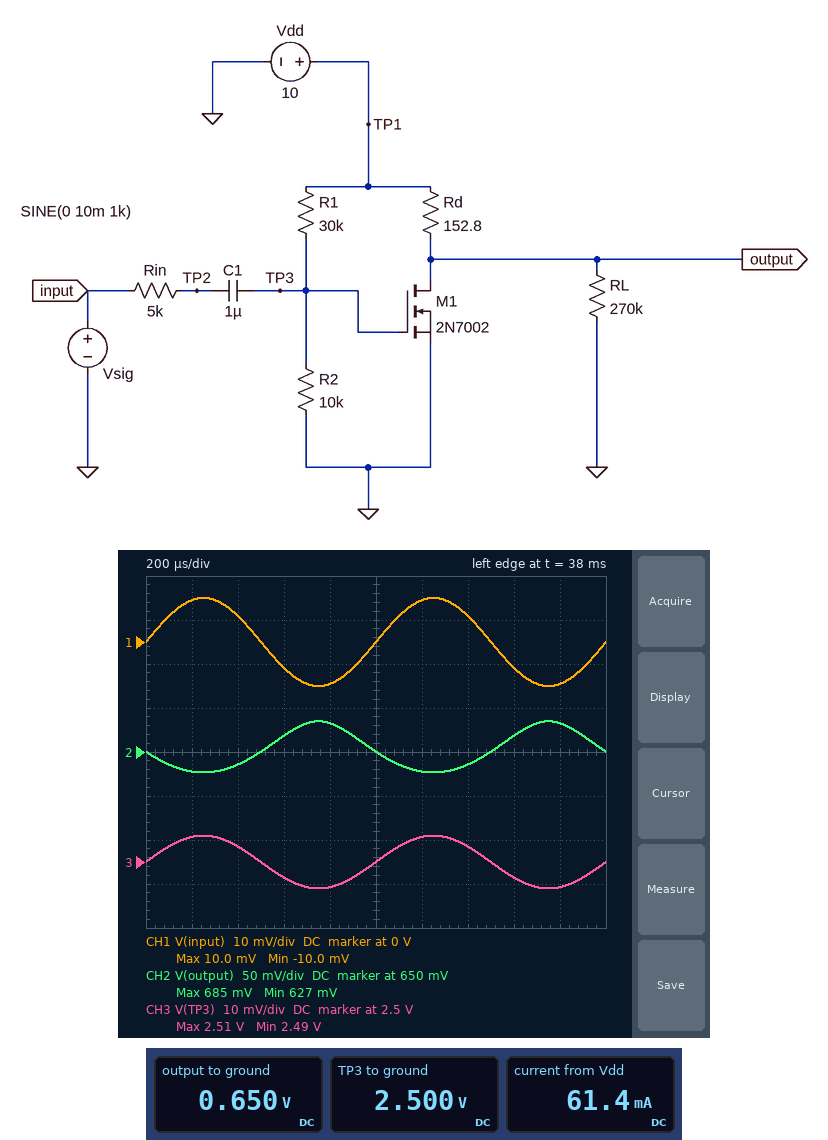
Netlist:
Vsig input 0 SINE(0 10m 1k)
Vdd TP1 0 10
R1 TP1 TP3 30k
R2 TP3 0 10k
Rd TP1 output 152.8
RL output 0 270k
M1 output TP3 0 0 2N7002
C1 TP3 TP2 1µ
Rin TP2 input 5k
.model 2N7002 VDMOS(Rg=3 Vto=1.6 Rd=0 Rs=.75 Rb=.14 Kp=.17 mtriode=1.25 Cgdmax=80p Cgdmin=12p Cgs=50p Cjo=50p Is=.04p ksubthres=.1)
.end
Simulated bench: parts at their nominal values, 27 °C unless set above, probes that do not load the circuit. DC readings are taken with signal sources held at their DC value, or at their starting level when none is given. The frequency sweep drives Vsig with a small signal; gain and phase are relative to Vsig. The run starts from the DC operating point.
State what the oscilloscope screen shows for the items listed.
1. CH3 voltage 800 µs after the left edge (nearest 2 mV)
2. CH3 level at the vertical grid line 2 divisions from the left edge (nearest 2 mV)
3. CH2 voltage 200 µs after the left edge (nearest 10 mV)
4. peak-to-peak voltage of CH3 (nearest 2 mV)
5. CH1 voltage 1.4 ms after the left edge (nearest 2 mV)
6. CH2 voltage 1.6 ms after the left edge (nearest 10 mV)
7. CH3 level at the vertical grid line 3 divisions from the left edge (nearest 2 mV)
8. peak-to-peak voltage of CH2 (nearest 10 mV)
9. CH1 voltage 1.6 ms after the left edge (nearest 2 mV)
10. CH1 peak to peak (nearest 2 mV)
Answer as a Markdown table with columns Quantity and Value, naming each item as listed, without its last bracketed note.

| Quantity | Value |
|---|---|
| CH3 voltage 800 µs after the left edge | 2.494 V |
| CH3 level at the vertical grid line 2 divisions from the left edge | 2.504 V |
| CH2 voltage 200 µs after the left edge | 630 mV |
| peak-to-peak voltage of CH3 | 12 mV |
| CH1 voltage 1.4 ms after the left edge | 6 mV |
| CH2 voltage 1.6 ms after the left edge | 670 mV |
| CH3 level at the vertical grid line 3 divisions from the left edge | 2.496 V |
| peak-to-peak voltage of CH2 | 60 mV |
| CH1 voltage 1.6 ms after the left edge | -6 mV |
| CH1 peak to peak | 20 mV |
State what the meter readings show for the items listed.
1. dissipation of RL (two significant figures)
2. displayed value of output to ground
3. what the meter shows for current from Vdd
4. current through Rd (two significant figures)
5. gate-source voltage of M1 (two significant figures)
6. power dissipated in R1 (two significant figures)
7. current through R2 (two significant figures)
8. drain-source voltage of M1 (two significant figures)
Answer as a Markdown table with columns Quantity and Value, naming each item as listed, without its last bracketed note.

| Quantity | Value |
|---|---|
| dissipation of RL | 1.6 µW |
| displayed value of output to ground | 0.650 V |
| what the meter shows for current from Vdd | 61.4 mA |
| current through Rd | 61 mA |
| gate-source voltage of M1 | 2.5 V |
| power dissipated in R1 | 1.9 mW |
| current through R2 | 250 µA |
| drain-source voltage of M1 | 650 mV |
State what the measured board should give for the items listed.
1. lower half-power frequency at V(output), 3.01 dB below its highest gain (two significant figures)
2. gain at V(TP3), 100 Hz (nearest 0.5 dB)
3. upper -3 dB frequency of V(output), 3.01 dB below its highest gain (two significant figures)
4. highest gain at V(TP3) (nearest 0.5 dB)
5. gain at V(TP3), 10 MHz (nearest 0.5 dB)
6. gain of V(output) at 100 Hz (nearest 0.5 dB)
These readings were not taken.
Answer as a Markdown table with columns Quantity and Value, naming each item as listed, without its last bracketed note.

| Quantity | Value |
|---|---|
| lower half-power frequency at V(output), 3.01 dB below its highest gain | 13 Hz |
| gain at V(TP3), 100 Hz | -4.5 dB |
| upper -3 dB frequency of V(output), 3.01 dB below its highest gain | 110 kHz |
| highest gain at V(TP3) | -4.5 dB |
| gain at V(TP3), 10 MHz | -43.0 dB |
| gain of V(output) at 100 Hz | 8.5 dB |
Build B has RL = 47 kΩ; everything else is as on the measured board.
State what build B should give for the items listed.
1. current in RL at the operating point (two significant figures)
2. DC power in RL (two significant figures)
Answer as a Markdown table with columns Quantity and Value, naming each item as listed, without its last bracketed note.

| Quantity | Value |
|---|---|
| current in RL at the operating point | 14 µA |
| DC power in RL | 9.0 µW |
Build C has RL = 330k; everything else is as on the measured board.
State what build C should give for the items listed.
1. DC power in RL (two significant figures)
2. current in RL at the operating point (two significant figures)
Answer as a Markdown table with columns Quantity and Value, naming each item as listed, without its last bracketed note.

| Quantity | Value |
|---|---|
| DC power in RL | 1.3 µW |
| current in RL at the operating point | 2.0 µA |
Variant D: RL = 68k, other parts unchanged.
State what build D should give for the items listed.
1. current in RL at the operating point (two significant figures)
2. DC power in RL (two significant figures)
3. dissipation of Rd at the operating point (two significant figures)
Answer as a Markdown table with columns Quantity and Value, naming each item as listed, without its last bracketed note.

| Quantity | Value |
|---|---|
| current in RL at the operating point | 9.6 µA |
| DC power in RL | 6.2 µW |
| dissipation of Rd at the operating point | 570 mW |
